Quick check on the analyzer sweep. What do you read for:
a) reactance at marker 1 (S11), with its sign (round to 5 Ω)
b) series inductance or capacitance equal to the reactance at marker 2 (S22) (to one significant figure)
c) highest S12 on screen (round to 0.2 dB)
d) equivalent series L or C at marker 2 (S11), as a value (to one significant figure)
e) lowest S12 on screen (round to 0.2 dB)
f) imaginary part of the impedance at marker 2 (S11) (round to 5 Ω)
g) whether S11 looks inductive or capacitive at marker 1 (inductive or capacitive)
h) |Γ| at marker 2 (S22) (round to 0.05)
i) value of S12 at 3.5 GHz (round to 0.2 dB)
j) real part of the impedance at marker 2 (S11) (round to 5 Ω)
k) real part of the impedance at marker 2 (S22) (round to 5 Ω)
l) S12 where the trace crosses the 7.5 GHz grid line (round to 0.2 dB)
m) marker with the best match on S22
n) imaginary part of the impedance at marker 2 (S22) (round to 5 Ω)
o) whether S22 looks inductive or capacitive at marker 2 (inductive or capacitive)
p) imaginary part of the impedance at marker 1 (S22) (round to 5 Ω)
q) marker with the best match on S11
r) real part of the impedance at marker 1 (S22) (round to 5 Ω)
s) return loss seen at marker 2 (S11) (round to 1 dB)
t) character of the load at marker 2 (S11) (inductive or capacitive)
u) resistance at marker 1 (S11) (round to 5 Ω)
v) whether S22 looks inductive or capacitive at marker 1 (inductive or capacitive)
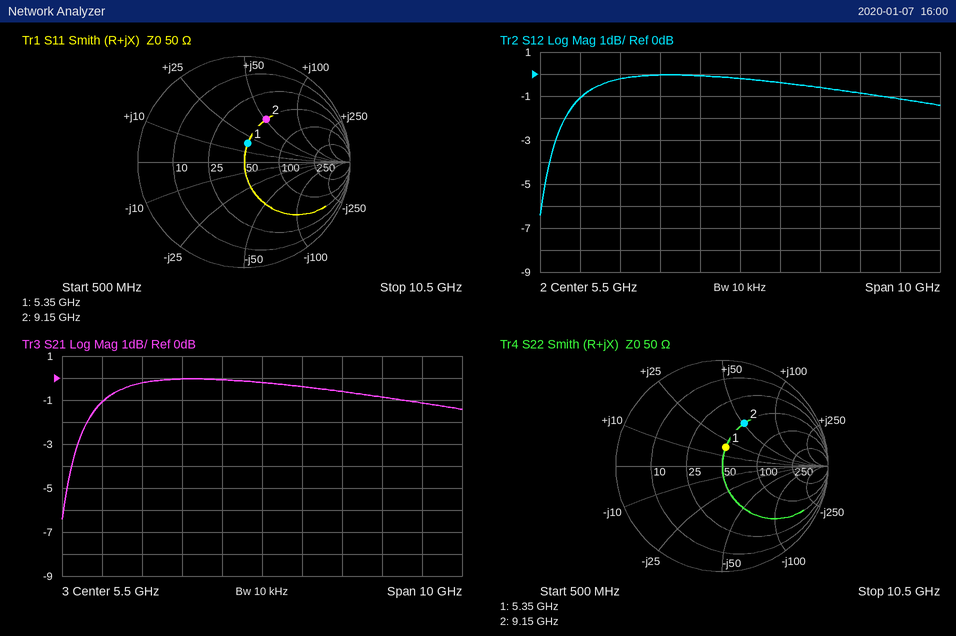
+20 Ω
900 pH
0.0 dB
900 pH
-6.4 dB
+50 Ω
inductive
0.45
0.0 dB
50 Ω
50 Ω
-0.6 dB
marker 1
+50 Ω
inductive
+20 Ω
marker 1
50 Ω
7 dB
inductive
50 Ω
inductive
